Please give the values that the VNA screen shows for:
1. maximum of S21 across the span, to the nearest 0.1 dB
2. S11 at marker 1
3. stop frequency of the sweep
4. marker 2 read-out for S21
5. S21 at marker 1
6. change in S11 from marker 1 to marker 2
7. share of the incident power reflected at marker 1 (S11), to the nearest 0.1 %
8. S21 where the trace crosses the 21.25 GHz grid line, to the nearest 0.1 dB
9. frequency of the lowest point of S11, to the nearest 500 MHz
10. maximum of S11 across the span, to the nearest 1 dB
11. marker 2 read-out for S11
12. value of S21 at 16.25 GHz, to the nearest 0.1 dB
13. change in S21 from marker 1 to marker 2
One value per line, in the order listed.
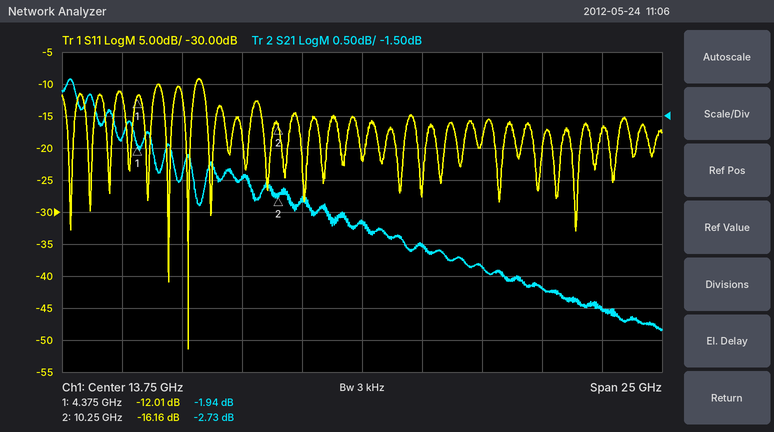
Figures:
-0.9 dB
-12.01 dB
26.25 GHz
-2.73 dB
-1.94 dB
-4.15 dB
6.3 %
-4.2 dB
6.5 GHz
-9 dB
-16.16 dB
-3.5 dB
-0.79 dB
